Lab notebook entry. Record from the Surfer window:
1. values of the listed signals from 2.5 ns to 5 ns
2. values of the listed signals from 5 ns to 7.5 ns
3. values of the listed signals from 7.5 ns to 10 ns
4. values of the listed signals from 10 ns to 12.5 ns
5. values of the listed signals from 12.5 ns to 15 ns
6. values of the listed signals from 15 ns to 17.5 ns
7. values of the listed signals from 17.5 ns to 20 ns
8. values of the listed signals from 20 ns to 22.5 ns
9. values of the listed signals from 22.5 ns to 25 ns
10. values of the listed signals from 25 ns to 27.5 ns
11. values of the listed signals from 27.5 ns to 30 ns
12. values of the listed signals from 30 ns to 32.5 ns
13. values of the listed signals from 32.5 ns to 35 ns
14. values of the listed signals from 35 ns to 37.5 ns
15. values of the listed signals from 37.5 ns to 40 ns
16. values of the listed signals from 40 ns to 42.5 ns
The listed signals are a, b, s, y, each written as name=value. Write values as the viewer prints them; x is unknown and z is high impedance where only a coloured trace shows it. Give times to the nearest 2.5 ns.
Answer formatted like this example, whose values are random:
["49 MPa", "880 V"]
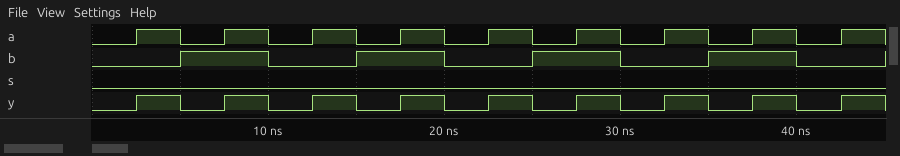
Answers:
["a=1, b=0, s=0, y=1", "a=0, b=1, s=0, y=0", "a=1, b=1, s=0, y=1", "a=0, b=0, s=0, y=0", "a=1, b=0, s=0, y=1", "a=0, b=1, s=0, y=0", "a=1, b=1, s=0, y=1", "a=0, b=0, s=0, y=0", "a=1, b=0, s=0, y=1", "a=0, b=1, s=0, y=0", "a=1, b=1, s=0, y=1", "a=0, b=0, s=0, y=0", "a=1, b=0, s=0, y=1", "a=0, b=1, s=0, y=0", "a=1, b=1, s=0, y=1", "a=0, b=0, s=0, y=0"]
